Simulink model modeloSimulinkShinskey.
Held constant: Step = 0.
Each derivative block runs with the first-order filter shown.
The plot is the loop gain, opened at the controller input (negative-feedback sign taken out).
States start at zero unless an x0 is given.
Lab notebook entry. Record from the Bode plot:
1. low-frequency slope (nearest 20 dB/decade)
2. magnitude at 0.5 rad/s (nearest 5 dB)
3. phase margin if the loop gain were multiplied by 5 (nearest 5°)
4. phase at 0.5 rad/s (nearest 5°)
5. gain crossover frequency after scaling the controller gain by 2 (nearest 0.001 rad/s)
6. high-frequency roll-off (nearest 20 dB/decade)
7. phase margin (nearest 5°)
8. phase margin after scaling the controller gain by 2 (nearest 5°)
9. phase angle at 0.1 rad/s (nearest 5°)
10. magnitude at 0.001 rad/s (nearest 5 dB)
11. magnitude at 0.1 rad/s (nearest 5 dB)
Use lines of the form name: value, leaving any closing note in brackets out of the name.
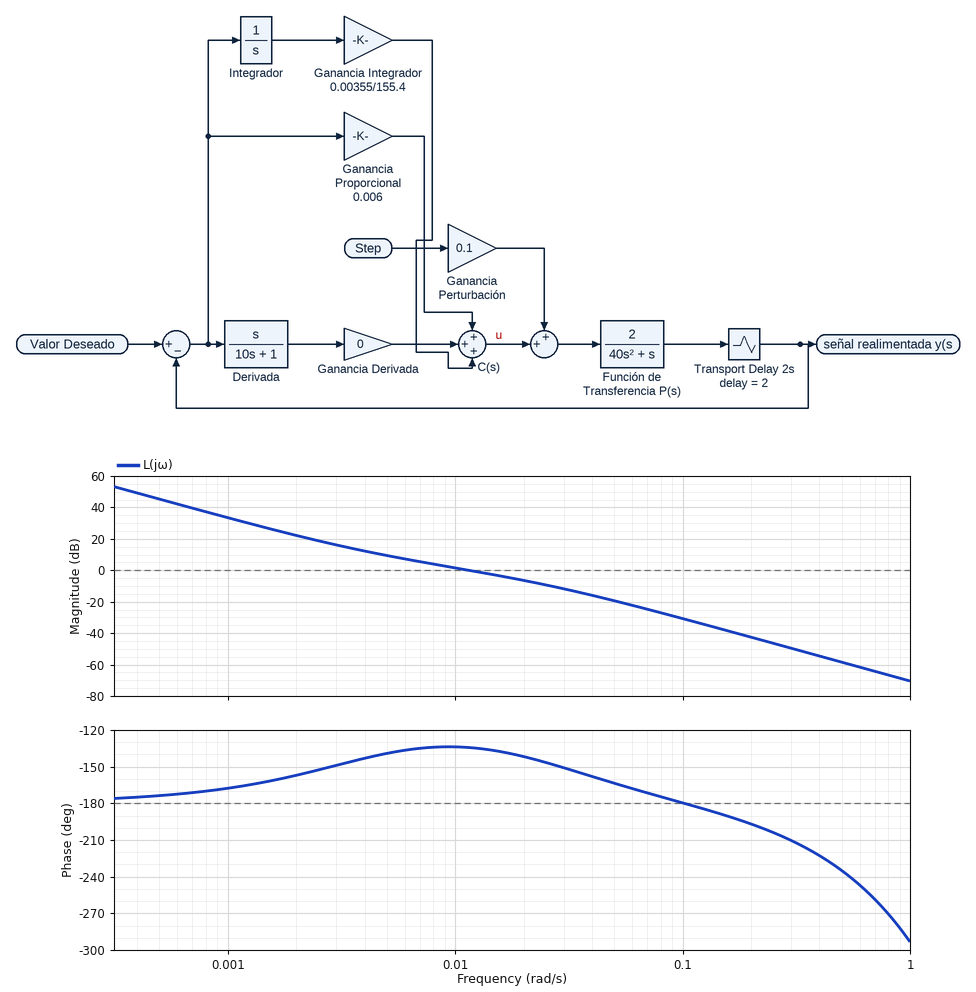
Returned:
low-frequency slope: -40 dB/decade
magnitude at 0.5 rad/s: -60 dB
phase margin if the loop gain were multiplied by 5: 25°
phase at 0.5 rad/s: -235°
gain crossover frequency after scaling the controller gain by 2: 0.019 rad/s
high-frequency roll-off: -40 dB/decade
phase margin: 45°
phase margin after scaling the controller gain by 2: 40°
phase angle at 0.1 rad/s: -180°
magnitude at 0.001 rad/s: 35 dB
magnitude at 0.1 rad/s: -30 dB
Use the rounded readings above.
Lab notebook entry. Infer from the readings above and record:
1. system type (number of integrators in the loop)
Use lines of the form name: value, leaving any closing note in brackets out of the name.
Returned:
system type: 2
